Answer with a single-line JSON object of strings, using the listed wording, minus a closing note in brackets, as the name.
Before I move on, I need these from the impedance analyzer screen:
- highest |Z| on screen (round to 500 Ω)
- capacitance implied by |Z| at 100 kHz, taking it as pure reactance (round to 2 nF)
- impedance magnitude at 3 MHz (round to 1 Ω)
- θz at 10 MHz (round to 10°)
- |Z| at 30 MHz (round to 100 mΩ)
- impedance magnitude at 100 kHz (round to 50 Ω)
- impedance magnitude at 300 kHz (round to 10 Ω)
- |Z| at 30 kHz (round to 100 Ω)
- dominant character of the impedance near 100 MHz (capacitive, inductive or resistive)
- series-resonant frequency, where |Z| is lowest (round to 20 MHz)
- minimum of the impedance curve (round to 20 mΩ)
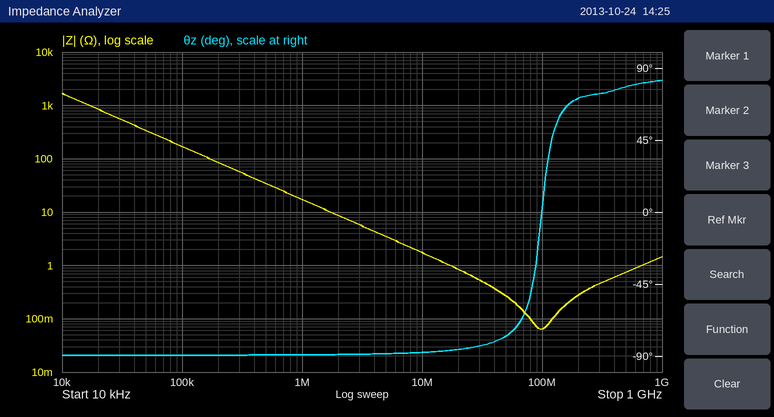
{"highest |Z| on screen": "1.5 kΩ", "capacitance implied by |Z| at 100 kHz, taking it as pure reactance": "10 nF", "impedance magnitude at 3 MHz": "6 Ω", "θz at 10 MHz": "-90°", "|Z| at 30 MHz": "500 mΩ", "impedance magnitude at 100 kHz": "150 Ω", "impedance magnitude at 300 kHz": "60 Ω", "|Z| at 30 kHz": "600 Ω", "dominant character of the impedance near 100 MHz": "resistive", "series-resonant frequency, where |Z| is lowest": "100 MHz", "minimum of the impedance curve": "60 mΩ"}
